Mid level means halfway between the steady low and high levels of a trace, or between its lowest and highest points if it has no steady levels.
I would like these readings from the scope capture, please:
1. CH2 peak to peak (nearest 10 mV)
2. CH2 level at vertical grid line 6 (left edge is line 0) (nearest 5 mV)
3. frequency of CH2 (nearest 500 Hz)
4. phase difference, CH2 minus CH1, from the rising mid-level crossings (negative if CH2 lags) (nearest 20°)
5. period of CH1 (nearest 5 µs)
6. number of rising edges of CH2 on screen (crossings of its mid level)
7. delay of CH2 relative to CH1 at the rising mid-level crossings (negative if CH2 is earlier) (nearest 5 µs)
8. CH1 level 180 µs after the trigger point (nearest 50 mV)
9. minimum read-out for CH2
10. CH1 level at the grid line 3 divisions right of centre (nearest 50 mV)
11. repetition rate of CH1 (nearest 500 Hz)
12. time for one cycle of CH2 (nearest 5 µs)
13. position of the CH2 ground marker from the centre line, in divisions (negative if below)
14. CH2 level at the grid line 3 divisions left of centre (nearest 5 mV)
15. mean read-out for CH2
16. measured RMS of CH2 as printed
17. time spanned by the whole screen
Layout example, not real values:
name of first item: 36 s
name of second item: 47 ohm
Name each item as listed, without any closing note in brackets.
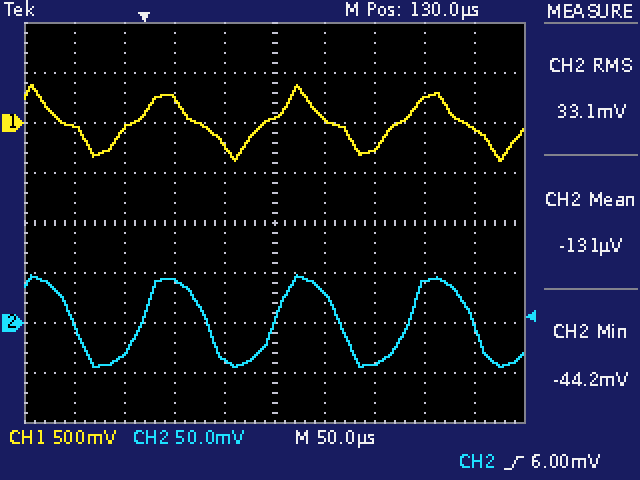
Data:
CH2 peak to peak: 90 mV
CH2 level at vertical grid line 6 (left edge is line 0): 30 mV
frequency of CH2: 7.5 kHz
phase difference, CH2 minus CH1, from the rising mid-level crossings (negative if CH2 lags): -20°
period of CH1: 135 µs
number of rising edges of CH2 on screen: 3
delay of CH2 relative to CH1 at the rising mid-level crossings (negative if CH2 is earlier): +10 µs
CH1 level 180 µs after the trigger point: 50 mV
minimum read-out for CH2: -44.2 mV
CH1 level at the grid line 3 divisions right of centre: 250 mV
repetition rate of CH1: 7.5 kHz
time for one cycle of CH2: 135 µs
position of the CH2 ground marker from the centre line, in divisions: -2.0 div
CH2 level at the grid line 3 divisions left of centre: -30 mV
mean read-out for CH2: -131 µV
measured RMS of CH2 as printed: 33.1 mV
time spanned by the whole screen: 500 µs
